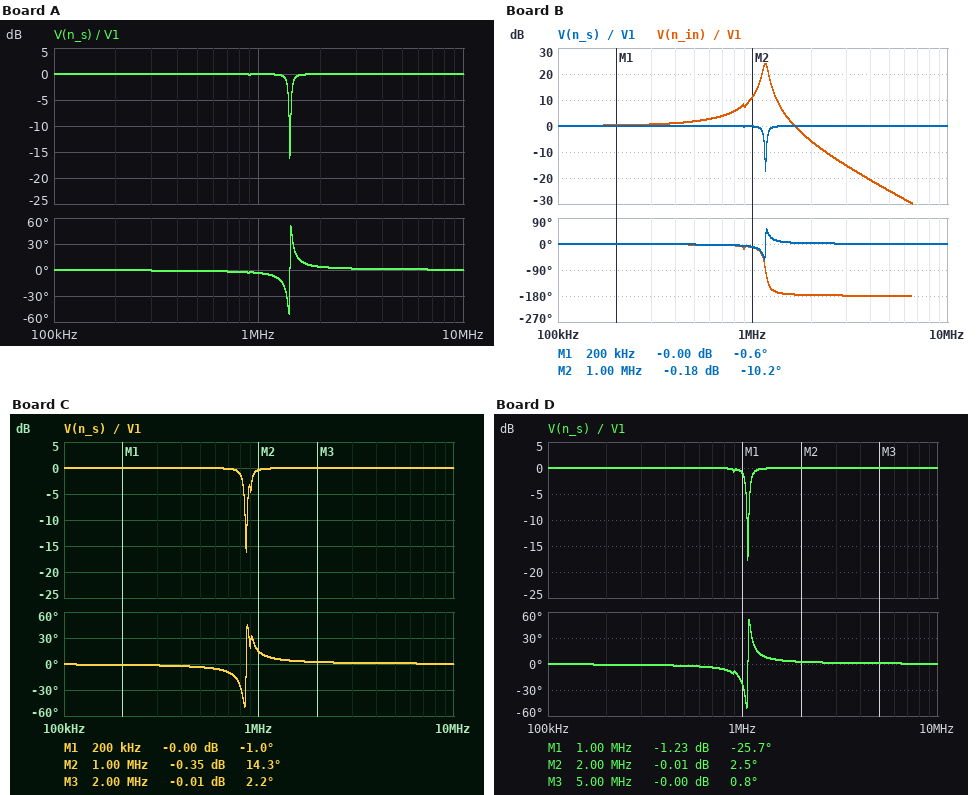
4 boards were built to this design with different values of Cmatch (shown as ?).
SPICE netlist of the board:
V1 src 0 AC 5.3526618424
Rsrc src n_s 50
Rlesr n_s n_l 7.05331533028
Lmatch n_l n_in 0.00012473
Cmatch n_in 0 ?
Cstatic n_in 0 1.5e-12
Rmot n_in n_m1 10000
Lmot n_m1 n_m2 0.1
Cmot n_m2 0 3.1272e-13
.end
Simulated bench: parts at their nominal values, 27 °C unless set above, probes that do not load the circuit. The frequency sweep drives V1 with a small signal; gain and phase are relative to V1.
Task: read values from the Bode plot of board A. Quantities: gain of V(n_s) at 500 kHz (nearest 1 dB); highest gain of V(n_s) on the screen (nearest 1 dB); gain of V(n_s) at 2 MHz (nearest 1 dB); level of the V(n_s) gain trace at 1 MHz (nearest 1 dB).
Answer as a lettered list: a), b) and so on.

a) 0 dB
b) 0 dB
c) 0 dB
d) 0 dB
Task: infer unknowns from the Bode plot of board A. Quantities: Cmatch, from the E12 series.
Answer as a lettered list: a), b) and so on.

a) 100 pF
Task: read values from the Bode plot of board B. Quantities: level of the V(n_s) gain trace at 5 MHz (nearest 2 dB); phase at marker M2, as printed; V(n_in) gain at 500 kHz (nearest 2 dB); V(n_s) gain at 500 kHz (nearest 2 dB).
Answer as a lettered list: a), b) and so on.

a) 0 dB
b) -10.2 deg
c) 2 dB
d) 0 dB
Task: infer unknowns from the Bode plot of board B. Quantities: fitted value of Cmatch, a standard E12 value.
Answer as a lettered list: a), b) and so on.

a) 150 pF
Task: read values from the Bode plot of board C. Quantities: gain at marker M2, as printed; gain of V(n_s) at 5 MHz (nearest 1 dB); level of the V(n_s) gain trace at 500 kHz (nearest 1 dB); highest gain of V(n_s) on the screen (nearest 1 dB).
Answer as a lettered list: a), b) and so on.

a) -0.35 dB
b) 0 dB
c) 0 dB
d) 0 dB
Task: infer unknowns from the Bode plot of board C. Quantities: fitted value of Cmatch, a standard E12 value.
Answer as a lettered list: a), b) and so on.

a) 270 pF
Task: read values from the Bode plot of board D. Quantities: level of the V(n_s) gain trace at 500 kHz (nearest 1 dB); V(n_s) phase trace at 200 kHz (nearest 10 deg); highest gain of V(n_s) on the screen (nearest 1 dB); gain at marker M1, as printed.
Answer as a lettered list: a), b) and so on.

a) 0 dB
b) 0 deg
c) 0 dB
d) -1.23 dB
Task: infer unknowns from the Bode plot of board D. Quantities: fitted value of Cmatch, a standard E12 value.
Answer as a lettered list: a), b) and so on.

a) 180 pF
